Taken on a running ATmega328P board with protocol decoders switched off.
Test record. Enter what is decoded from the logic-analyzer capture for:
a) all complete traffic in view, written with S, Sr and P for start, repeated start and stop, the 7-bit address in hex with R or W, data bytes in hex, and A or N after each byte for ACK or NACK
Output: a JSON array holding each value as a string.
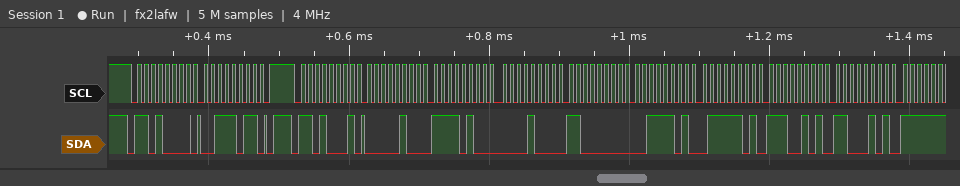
["S 68W A 3B A P S 68R A 04 A F4 A 08 A C0 A 3D A 7D A E5 A C5 A"]
